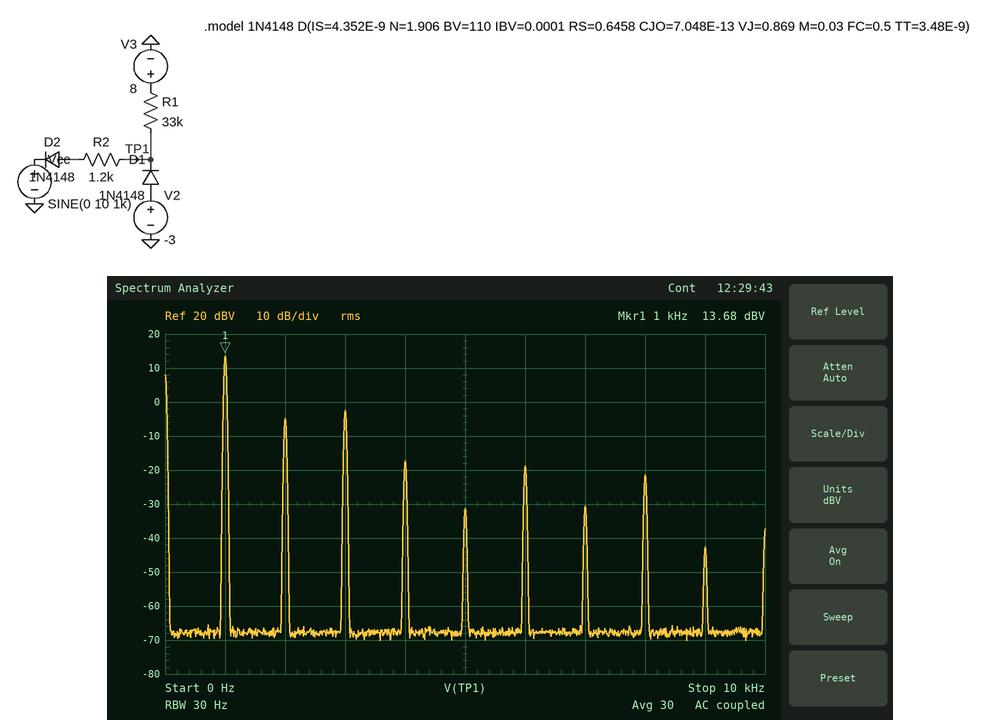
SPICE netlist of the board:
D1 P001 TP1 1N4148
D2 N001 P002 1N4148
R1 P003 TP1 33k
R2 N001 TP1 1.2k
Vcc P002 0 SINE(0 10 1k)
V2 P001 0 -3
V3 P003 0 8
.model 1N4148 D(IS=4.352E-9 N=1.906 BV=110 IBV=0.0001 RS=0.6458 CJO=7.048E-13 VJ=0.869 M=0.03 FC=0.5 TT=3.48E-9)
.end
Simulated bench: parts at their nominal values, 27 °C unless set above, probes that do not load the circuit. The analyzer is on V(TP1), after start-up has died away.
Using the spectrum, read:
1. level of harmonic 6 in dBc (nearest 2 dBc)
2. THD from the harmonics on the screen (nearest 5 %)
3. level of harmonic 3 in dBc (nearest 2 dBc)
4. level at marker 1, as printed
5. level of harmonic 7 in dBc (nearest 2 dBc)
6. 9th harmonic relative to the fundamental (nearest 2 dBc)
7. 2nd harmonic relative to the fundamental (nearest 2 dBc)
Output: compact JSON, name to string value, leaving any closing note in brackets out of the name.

{"level of harmonic 6 in dBc": "-32 dBc", "THD from the harmonics on the screen": "20 %", "level of harmonic 3 in dBc": "-16 dBc", "level at marker 1, as printed": "13.68 dBV", "level of harmonic 7 in dBc": "-44 dBc", "9th harmonic relative to the fundamental": "-56 dBc", "2nd harmonic relative to the fundamental": "-18 dBc"}
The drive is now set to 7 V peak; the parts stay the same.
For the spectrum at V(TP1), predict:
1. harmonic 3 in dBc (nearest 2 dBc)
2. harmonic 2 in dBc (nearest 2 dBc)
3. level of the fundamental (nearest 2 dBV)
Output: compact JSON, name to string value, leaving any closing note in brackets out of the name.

{"harmonic 3 in dBc": "-24 dBc", "harmonic 2 in dBc": "-20 dBc", "level of the fundamental": "12 dBV"}
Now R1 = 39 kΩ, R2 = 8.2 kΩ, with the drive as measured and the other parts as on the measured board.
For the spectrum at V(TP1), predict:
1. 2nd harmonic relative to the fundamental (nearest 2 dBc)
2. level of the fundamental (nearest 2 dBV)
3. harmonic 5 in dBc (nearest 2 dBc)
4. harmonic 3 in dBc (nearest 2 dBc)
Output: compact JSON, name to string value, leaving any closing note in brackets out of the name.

{"2nd harmonic relative to the fundamental": "-28 dBc", "level of the fundamental": "14 dBV", "harmonic 5 in dBc": "-34 dBc", "harmonic 3 in dBc": "-18 dBc"}
